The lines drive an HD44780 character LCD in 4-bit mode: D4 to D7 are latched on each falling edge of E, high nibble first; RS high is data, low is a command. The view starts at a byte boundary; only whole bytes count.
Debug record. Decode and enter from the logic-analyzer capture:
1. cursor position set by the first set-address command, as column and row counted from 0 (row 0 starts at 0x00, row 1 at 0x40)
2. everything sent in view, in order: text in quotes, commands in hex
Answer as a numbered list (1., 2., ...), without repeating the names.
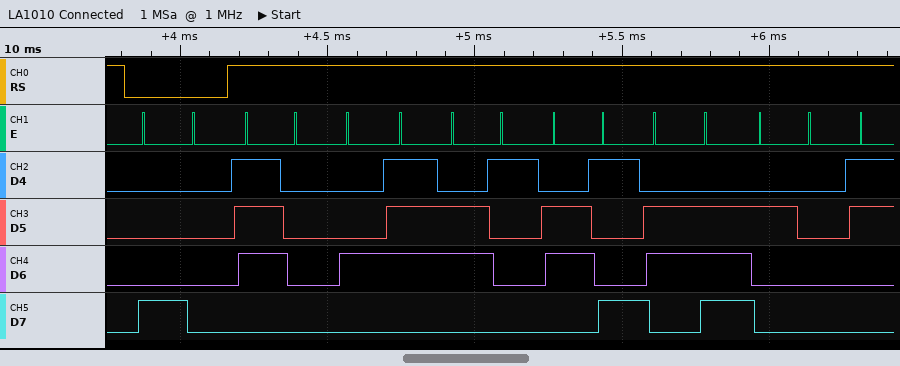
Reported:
1. column 0, row 0
2. 0x80 "pGain "
